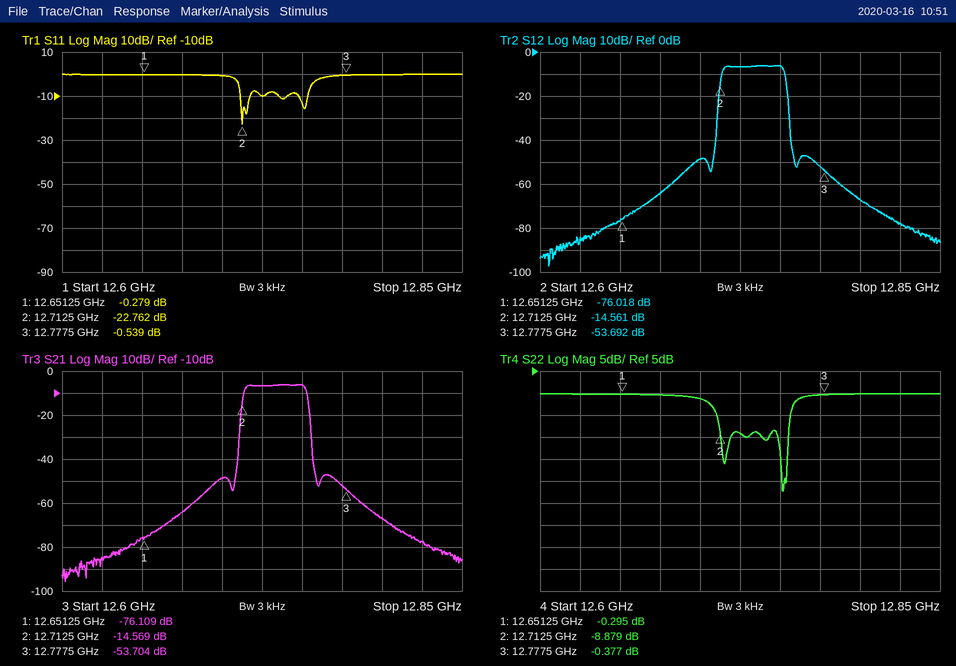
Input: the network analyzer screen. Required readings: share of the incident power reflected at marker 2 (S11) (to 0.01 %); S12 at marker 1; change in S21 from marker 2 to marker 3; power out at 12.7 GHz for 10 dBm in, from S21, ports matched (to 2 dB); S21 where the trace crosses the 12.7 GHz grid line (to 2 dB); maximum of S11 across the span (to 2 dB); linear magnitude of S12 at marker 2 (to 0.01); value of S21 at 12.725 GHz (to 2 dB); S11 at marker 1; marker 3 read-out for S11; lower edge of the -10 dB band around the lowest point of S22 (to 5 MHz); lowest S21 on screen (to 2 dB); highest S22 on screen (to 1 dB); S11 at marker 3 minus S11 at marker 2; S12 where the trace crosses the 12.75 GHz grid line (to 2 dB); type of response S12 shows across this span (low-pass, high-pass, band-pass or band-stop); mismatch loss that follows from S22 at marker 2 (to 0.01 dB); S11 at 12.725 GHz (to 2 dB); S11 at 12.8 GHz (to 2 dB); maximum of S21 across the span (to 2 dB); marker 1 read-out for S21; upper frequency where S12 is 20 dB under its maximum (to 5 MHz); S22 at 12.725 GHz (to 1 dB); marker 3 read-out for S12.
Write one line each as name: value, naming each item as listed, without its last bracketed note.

share of the incident power reflected at marker 2 (S11): 0.53 %
S12 at marker 1: -76.018 dB
change in S21 from marker 2 to marker 3: -39.135 dB
power out at 12.7 GHz for 10 dBm in, from S21, ports matched: -38 dBm
S21 where the trace crosses the 12.7 GHz grid line: -48 dB
maximum of S11 across the span: 0 dB
linear magnitude of S12 at marker 2: 0.19
value of S21 at 12.725 GHz: -6 dB
S11 at marker 1: -0.279 dB
marker 3 read-out for S11: -0.539 dB
lower edge of the -10 dB band around the lowest point of S22: 12.750 GHz
lowest S21 on screen: -96 dB
highest S22 on screen: 0 dB
S11 at marker 3 minus S11 at marker 2: 22.223 dB
S12 where the trace crosses the 12.75 GHz grid line: -6 dB
type of response S12 shows across this span: band-pass
mismatch loss that follows from S22 at marker 2: 0.60 dB
S11 at 12.725 GHz: -10 dB
S11 at 12.8 GHz: 0 dB
maximum of S21 across the span: -6 dB
marker 1 read-out for S21: -76.109 dB
upper frequency where S12 is 20 dB under its maximum: 12.755 GHz
S22 at 12.725 GHz: -9 dB
marker 3 read-out for S12: -53.692 dB
